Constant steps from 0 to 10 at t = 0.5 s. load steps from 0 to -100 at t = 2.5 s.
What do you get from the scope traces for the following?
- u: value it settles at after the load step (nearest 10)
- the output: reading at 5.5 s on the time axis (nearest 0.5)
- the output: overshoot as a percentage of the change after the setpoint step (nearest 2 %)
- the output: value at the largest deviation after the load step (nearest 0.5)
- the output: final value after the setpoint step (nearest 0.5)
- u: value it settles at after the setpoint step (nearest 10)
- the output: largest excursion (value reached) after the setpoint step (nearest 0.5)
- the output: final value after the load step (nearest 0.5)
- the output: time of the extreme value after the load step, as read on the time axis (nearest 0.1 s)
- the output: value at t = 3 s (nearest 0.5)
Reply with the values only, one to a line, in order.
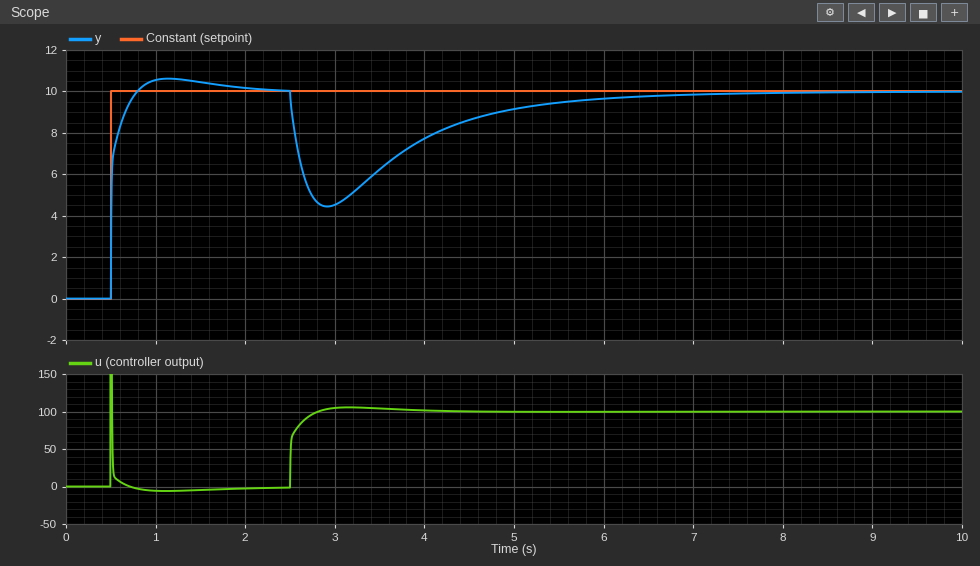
100
9.5
6 %
4.5
10.0
0
10.5
10.0
2.9 s
4.5
